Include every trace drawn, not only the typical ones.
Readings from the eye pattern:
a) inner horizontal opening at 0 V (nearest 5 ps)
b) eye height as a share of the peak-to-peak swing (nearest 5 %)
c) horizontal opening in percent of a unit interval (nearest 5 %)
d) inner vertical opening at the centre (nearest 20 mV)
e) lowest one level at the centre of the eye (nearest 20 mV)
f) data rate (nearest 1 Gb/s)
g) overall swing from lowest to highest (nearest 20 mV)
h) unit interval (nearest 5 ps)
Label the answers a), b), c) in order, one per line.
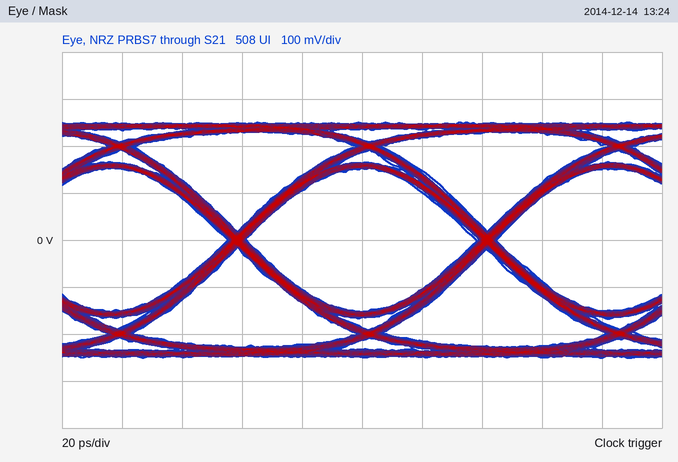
a) 75 ps
b) 60 %
c) 90 %
d) 300 mV
e) 160 mV
f) 12 Gb/s
g) 500 mV
h) 85 ps
